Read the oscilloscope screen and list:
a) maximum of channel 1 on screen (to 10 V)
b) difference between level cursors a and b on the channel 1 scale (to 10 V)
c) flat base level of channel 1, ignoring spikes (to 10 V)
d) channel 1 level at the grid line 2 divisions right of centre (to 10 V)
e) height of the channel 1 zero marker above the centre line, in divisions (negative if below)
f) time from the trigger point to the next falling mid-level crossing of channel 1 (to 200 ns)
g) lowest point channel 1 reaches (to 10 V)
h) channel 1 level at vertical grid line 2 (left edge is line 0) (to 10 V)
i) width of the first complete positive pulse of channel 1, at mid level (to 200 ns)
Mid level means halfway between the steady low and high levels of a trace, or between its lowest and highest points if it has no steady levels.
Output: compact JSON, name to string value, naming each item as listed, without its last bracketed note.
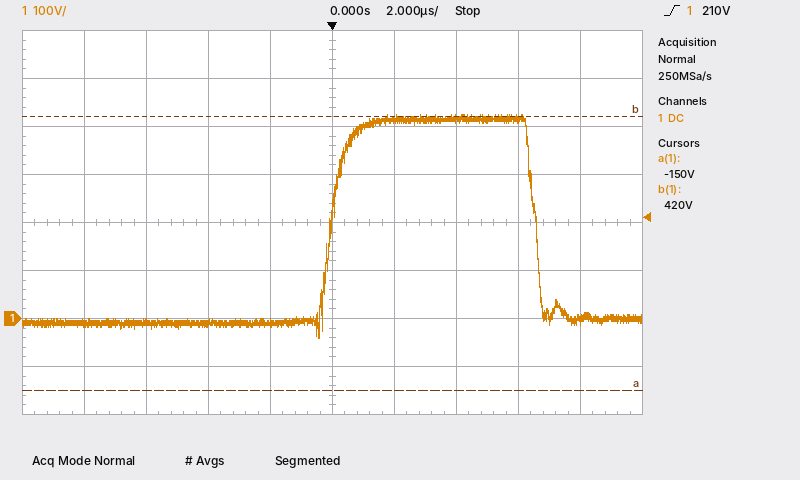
{"maximum of channel 1 on screen": "420 V", "difference between level cursors a and b on the channel 1 scale": "570 V", "flat base level of channel 1, ignoring spikes": "-10 V", "channel 1 level at the grid line 2 divisions right of centre": "420 V", "height of the channel 1 zero marker above the centre line, in divisions": "-2.0 div", "time from the trigger point to the next falling mid-level crossing of channel 1": "6.6 µs", "lowest point channel 1 reaches": "-40 V", "channel 1 level at vertical grid line 2 (left edge is line 0)": "-10 V", "width of the first complete positive pulse of channel 1, at mid level": "6.6 µs"}
